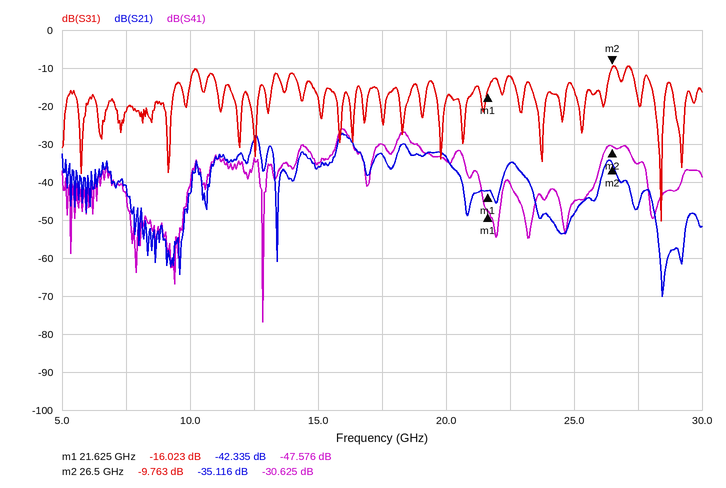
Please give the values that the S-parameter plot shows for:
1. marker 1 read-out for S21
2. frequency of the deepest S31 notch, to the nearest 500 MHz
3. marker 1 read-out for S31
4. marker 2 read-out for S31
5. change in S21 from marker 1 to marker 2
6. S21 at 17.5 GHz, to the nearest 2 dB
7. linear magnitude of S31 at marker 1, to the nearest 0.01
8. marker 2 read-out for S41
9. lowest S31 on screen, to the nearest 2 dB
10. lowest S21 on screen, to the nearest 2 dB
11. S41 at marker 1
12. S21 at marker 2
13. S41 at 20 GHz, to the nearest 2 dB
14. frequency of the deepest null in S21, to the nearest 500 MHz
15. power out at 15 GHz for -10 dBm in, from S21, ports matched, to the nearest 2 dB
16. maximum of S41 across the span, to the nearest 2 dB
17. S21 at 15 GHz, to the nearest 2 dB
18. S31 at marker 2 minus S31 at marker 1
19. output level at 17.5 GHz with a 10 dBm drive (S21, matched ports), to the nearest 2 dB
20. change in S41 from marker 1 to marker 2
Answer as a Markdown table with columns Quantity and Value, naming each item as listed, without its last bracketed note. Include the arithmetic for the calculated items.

| Quantity | Value |
|---|---|
| marker 1 read-out for S21 | -42.335 dB |
| frequency of the deepest S31 notch, to the nearest 500 MHz | 28.5 GHz |
| marker 1 read-out for S31 | -16.023 dB |
| marker 2 read-out for S31 | -9.763 dB |
| change in S21 from marker 1 to marker 2 | -35.116 − (-42.335) = 7.219 dB |
| S21 at 17.5 GHz, to the nearest 2 dB | -32 dB |
| linear magnitude of S31 at marker 1, to the nearest 0.01 | 10^(-16.023/20) ≈ 0.16 |
| marker 2 read-out for S41 | -30.625 dB |
| lowest S31 on screen, to the nearest 2 dB | -50 dB |
| lowest S21 on screen, to the nearest 2 dB | -70 dB |
| S41 at marker 1 | -47.576 dB |
| S21 at marker 2 | -35.116 dB |
| S41 at 20 GHz, to the nearest 2 dB | -34 dB |
| frequency of the deepest null in S21, to the nearest 500 MHz | 28.5 GHz |
| power out at 15 GHz for -10 dBm in, from S21, ports matched, to the nearest 2 dB | -10 dBm + (-36 dB) = -46 dBm |
| maximum of S41 across the span, to the nearest 2 dB | -26 dB |
| S21 at 15 GHz, to the nearest 2 dB | -36 dB |
| S31 at marker 2 minus S31 at marker 1 | -9.763 − (-16.023) = 6.260 dB |
| output level at 17.5 GHz with a 10 dBm drive (S21, matched ports), to the nearest 2 dB | 10 dBm + (-32 dB) = -22 dBm |
| change in S41 from marker 1 to marker 2 | -30.625 − (-47.576) = 16.951 dB |
